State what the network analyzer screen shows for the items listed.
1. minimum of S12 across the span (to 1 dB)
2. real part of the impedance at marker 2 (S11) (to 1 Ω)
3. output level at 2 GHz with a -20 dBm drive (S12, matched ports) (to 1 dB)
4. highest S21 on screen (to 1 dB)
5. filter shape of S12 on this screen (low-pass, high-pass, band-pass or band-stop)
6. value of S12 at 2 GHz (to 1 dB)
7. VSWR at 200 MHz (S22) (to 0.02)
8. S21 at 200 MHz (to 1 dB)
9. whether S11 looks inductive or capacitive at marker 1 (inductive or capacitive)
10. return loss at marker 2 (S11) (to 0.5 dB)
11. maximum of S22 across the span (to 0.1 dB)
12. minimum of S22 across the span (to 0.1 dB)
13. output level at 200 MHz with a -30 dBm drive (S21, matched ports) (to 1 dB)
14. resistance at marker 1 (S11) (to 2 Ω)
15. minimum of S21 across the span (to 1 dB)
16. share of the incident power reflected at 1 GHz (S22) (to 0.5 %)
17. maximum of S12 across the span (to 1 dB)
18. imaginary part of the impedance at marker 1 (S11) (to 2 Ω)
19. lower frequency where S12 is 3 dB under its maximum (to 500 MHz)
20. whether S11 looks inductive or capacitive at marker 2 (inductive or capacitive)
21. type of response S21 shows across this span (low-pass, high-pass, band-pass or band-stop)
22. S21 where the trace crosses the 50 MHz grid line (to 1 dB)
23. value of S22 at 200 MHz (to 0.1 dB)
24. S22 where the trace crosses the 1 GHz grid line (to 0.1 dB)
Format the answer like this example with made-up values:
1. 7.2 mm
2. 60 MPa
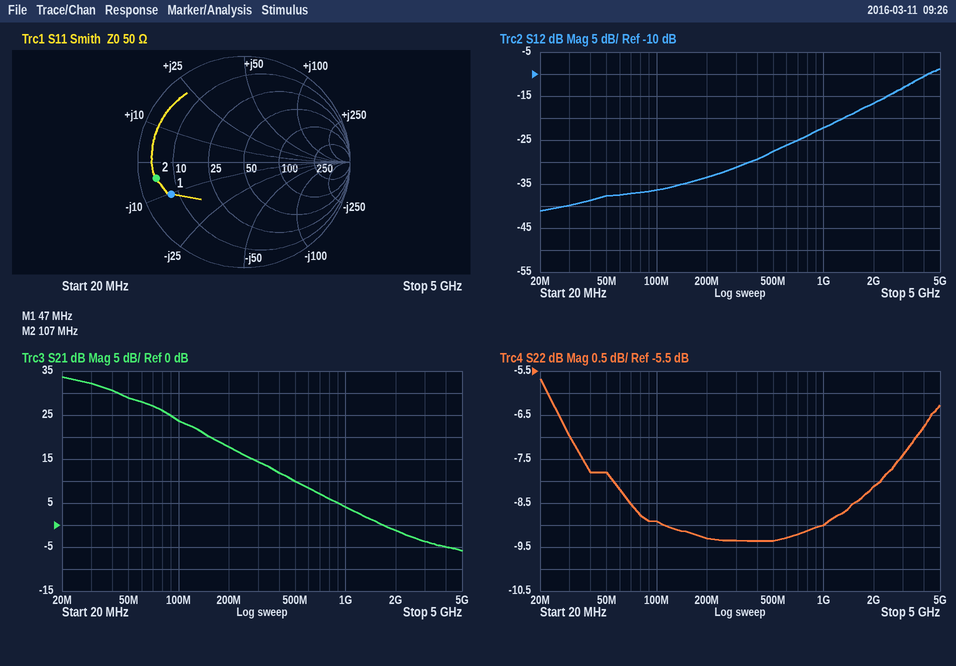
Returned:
1. -41 dB
2. 4 Ω
3. -37 dBm
4. 34 dB
5. high-pass
6. -17 dB
7. 2.04
8. 18 dB
9. capacitive
10. 1.5 dB
11. -5.7 dB
12. -9.4 dB
13. -12 dBm
14. 8 Ω
15. -6 dB
16. 12.5 %
17. -9 dB
18. -10 Ω
19. 3.5 GHz
20. capacitive
21. low-pass
22. 29 dB
23. -9.3 dB
24. -9.0 dB
